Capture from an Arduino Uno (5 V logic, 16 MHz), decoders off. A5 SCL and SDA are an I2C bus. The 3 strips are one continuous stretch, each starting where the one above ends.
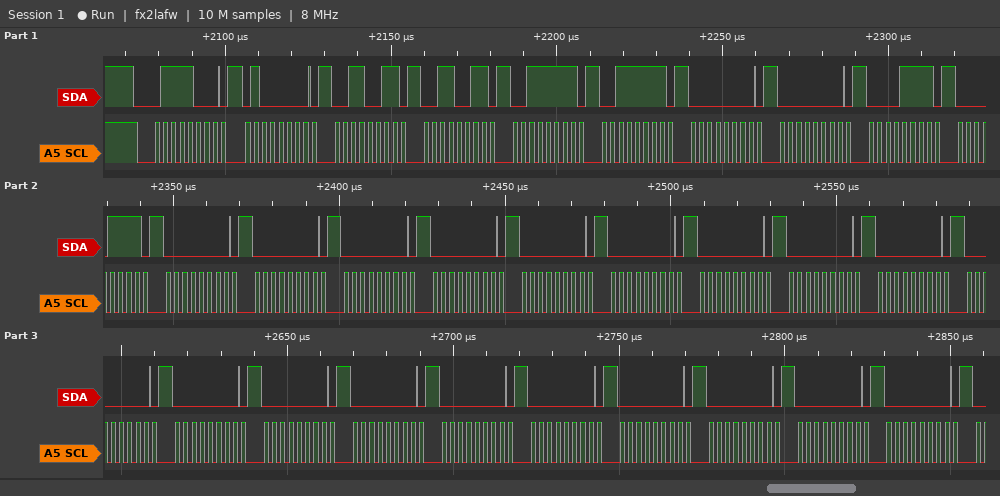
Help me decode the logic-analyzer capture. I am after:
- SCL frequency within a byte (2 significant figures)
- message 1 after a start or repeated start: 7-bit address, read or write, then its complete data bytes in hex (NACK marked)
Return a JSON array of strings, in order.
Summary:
["400 kHz", "0x3C write: 40 33 33 3F 3F 00 00 0F 0F 00 00 00 00 00 00 00 00 00 00 00 00 00 00 00 00 00 00 00"]
